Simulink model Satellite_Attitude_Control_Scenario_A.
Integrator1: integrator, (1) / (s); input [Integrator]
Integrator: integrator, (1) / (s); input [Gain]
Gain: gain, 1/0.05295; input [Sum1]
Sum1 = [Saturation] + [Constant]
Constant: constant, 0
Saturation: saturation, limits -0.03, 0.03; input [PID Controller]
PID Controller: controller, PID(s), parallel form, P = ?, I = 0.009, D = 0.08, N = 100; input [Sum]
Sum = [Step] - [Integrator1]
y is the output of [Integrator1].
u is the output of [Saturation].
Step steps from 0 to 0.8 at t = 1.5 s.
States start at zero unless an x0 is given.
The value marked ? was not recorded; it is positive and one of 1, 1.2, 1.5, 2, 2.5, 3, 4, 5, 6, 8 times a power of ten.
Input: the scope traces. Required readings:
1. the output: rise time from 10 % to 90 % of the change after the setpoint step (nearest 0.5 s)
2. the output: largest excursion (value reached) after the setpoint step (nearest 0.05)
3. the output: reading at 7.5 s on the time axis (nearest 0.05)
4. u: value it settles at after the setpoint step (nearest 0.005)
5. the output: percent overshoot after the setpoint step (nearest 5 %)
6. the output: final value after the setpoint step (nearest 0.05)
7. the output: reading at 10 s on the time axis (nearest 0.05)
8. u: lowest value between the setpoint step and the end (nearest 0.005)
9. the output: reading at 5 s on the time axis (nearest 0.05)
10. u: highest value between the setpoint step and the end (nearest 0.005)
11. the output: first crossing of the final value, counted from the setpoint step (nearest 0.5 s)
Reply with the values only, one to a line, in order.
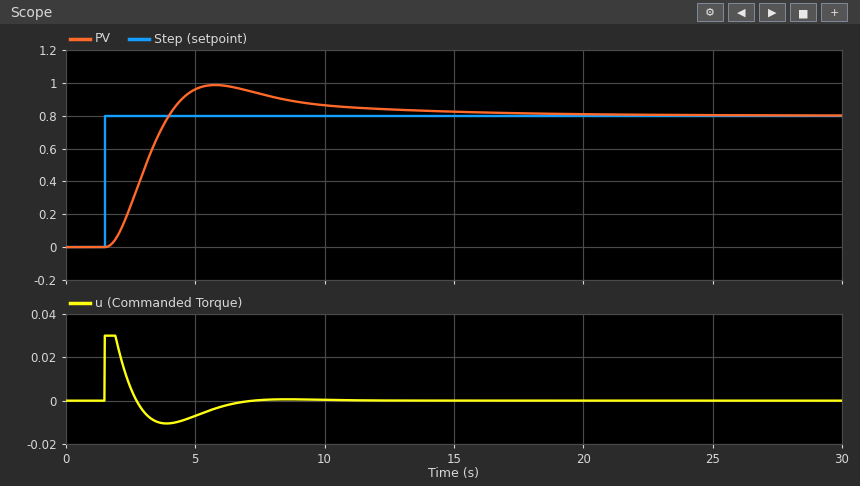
1.5 s
1.00
0.95
0.000
25 %
0.80
0.85
-0.010
0.95
0.030
2.5 s
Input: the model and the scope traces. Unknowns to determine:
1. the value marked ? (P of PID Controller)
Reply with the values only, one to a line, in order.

0.06
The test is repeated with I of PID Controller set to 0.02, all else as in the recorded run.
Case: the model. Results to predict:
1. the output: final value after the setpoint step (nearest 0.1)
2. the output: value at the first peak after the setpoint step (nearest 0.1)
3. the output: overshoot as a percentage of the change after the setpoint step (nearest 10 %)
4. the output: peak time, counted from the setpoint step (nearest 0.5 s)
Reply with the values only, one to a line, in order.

0.8
1.1
40 %
4.0 s
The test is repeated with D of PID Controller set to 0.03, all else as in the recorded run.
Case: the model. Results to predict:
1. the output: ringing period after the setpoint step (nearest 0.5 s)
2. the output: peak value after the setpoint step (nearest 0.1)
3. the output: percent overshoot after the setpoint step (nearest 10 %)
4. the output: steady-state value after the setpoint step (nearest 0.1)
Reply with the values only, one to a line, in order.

6.0 s
1.3
60 %
0.8
